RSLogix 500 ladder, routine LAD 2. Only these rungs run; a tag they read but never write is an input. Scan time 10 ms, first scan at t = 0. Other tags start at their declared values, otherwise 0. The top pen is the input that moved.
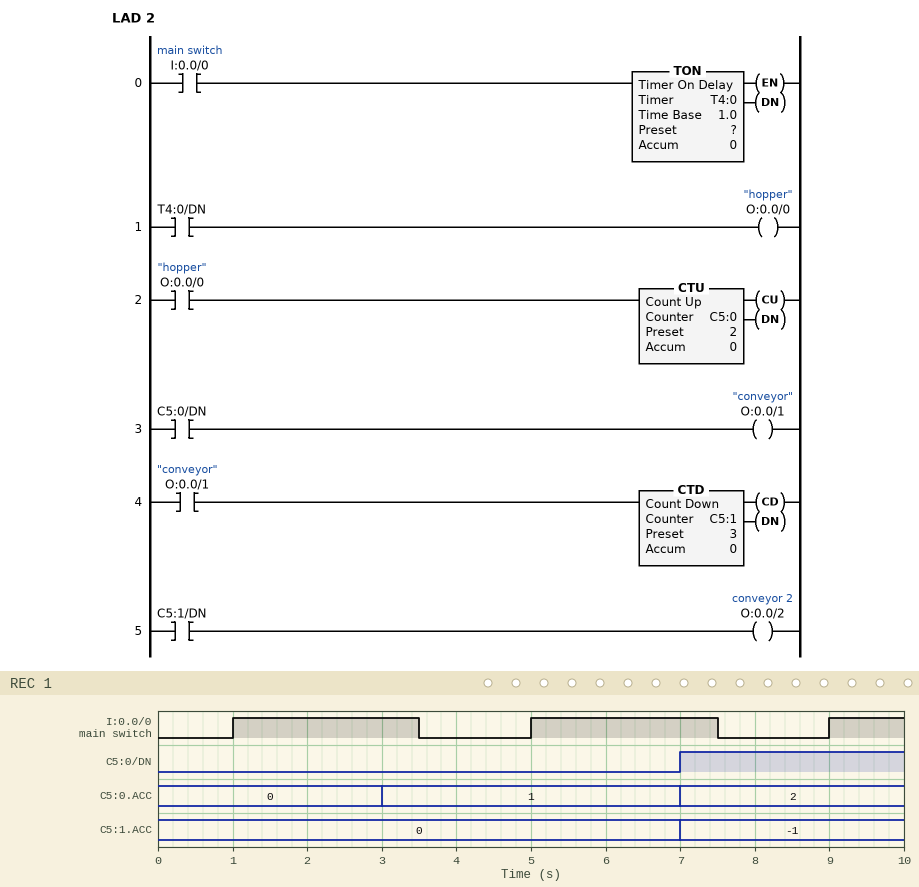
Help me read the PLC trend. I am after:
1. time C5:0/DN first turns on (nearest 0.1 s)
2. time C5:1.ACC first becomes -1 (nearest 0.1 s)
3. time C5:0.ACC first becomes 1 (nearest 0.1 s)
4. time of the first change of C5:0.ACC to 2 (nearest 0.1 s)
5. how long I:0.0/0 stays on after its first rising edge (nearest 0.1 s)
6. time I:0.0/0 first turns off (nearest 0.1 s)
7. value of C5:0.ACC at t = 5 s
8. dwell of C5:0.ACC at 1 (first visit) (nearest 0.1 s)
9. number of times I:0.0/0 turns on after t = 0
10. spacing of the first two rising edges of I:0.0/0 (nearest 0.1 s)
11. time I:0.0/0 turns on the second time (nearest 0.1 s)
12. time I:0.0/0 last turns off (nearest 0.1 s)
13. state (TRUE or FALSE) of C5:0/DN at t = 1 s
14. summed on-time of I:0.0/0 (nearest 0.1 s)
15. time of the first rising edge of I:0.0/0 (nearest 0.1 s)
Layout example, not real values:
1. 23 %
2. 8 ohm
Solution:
1. 7.0 s
2. 7.0 s
3. 3.0 s
4. 7.0 s
5. 2.5 s
6. 3.5 s
7. 1
8. 4.0 s
9. 3
10. 4.0 s
11. 5.0 s
12. 7.5 s
13. FALSE
14. 6.0 s
15. 1.0 s
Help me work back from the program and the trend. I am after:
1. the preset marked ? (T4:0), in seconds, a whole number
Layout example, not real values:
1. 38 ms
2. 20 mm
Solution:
1. 2 s
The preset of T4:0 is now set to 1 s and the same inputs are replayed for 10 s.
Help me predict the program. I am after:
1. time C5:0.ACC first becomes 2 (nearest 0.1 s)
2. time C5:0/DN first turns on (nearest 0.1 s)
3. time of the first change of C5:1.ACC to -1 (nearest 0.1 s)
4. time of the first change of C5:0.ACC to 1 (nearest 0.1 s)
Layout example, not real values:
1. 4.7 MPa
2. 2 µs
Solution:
1. 6.0 s
2. 6.0 s
3. 6.0 s
4. 2.0 s
